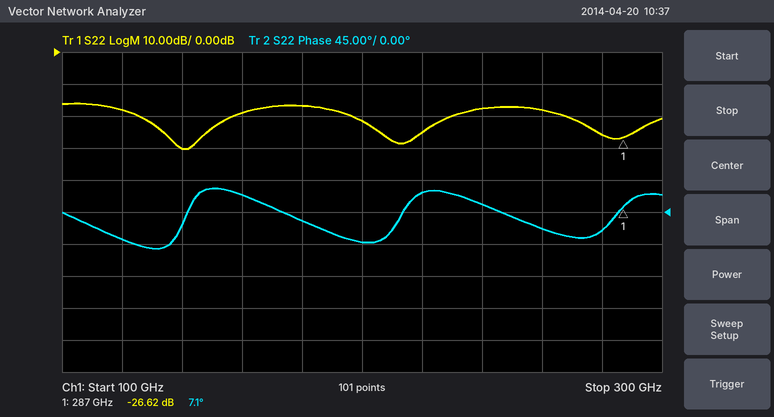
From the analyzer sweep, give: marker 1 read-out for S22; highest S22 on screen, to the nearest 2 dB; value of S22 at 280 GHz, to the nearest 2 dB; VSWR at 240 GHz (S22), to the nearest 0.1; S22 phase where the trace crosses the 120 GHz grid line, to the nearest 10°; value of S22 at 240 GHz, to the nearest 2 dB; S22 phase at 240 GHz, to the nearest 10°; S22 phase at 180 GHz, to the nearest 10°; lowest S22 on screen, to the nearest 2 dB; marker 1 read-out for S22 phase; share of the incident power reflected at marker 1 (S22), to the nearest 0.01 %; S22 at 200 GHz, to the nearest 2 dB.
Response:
-26.62 dB
-16 dB
-26 dB
1.3
-40°
-18 dB
10°
-10°
-30 dB
7.1°
0.22 %
-22 dB
